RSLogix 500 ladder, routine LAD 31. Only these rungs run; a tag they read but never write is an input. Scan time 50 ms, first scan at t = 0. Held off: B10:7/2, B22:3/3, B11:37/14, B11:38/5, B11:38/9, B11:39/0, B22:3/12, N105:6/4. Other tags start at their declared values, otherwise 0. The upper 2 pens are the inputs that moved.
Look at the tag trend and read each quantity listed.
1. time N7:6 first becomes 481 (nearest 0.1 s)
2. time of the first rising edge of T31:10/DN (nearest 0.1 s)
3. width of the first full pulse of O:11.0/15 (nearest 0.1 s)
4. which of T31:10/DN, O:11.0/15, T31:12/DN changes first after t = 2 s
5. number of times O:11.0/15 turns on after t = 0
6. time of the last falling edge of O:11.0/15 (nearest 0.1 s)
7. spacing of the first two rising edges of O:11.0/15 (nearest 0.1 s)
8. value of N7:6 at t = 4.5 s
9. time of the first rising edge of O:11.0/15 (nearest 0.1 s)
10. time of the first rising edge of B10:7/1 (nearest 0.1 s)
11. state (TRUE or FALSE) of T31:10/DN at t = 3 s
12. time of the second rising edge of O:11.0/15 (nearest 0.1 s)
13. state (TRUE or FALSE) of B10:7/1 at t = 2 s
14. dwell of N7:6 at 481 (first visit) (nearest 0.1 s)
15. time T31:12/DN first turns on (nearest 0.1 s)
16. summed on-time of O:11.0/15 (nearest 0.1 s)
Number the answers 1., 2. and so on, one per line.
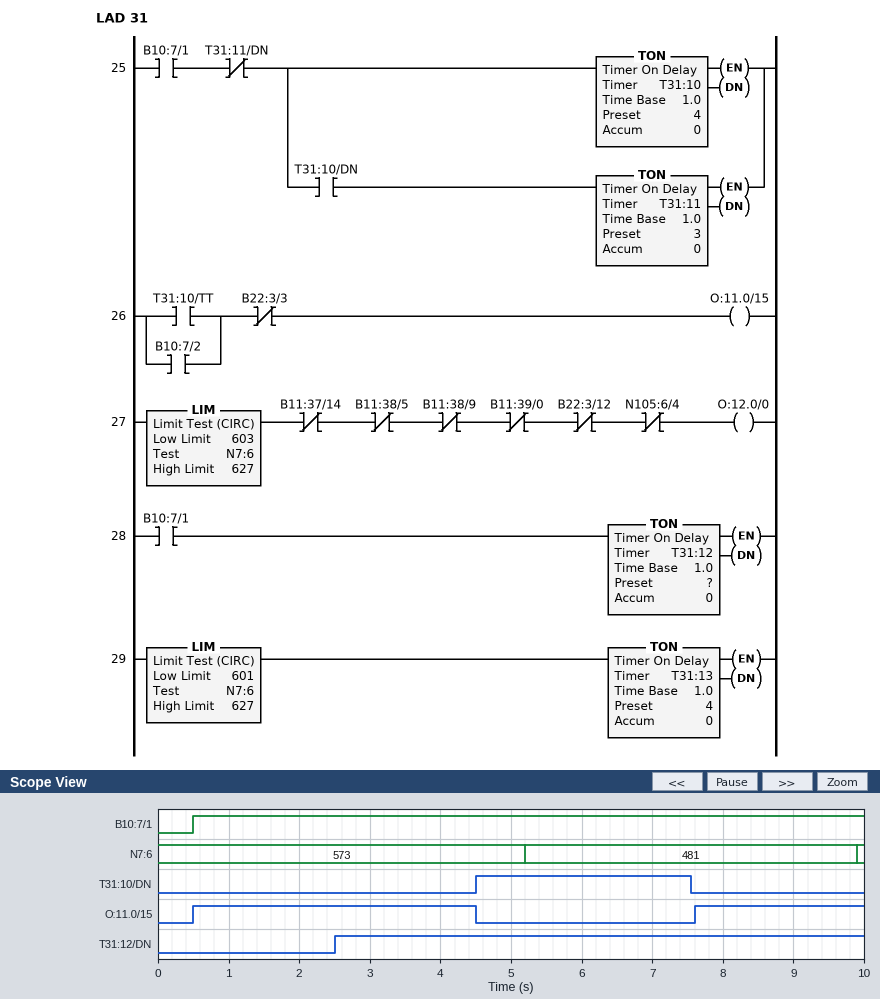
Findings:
1. 5.2 s
2. 4.5 s
3. 4.0 s
4. T31:12/DN
5. 2
6. 4.5 s
7. 7.1 s
8. 573
9. 0.5 s
10. 0.5 s
11. FALSE
12. 7.6 s
13. TRUE
14. 4.7 s
15. 2.5 s
16. 6.4 s
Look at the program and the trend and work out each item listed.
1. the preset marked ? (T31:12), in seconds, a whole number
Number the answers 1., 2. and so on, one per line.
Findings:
1. 2 s
